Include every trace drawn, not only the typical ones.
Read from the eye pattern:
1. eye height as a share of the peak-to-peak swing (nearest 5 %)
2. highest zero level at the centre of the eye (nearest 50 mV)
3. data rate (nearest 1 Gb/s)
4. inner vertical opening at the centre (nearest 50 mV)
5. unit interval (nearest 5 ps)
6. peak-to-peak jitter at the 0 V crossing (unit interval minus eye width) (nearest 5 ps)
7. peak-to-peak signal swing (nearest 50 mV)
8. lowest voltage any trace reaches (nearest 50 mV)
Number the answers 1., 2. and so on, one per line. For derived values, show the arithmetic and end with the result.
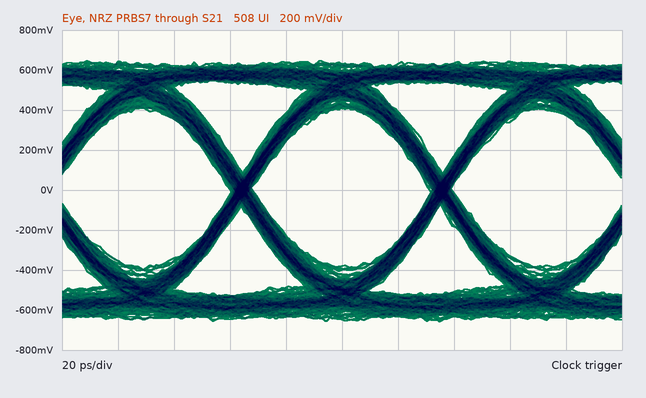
1. 800 mV / 1.30 V ≈ 61.5 %, so 60 % to the nearest 5 %
2. -400 mV
3. 14 Gb/s
4. 800 mV
5. 70 ps
6. 10 ps
7. 1.30 V
8. -650 mV
